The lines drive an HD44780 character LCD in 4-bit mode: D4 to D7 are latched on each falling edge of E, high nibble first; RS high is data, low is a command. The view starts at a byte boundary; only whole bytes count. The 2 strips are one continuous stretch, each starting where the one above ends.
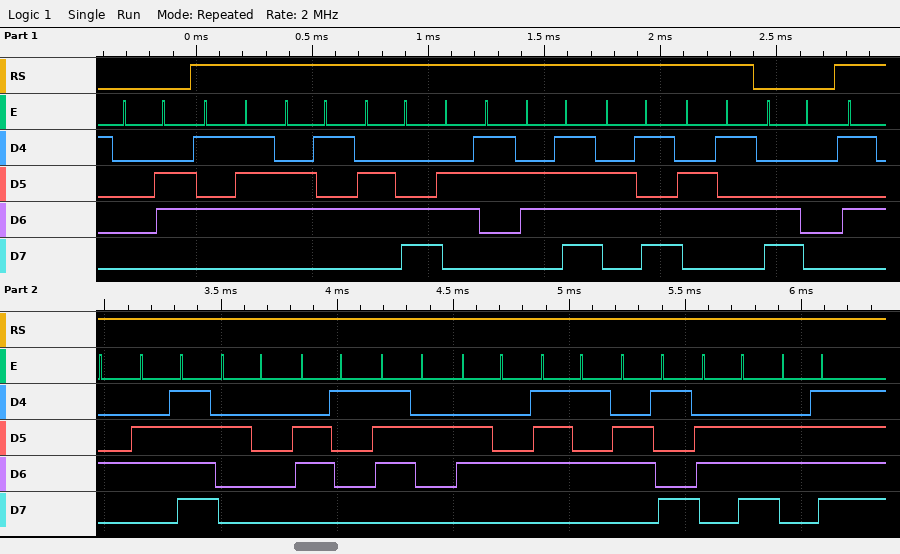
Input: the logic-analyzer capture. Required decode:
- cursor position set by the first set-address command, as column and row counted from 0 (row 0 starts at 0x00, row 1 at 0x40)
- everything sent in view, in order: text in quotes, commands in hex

column 0, row 1
0x06 "Welcome" 0xC0 "To arduino"
